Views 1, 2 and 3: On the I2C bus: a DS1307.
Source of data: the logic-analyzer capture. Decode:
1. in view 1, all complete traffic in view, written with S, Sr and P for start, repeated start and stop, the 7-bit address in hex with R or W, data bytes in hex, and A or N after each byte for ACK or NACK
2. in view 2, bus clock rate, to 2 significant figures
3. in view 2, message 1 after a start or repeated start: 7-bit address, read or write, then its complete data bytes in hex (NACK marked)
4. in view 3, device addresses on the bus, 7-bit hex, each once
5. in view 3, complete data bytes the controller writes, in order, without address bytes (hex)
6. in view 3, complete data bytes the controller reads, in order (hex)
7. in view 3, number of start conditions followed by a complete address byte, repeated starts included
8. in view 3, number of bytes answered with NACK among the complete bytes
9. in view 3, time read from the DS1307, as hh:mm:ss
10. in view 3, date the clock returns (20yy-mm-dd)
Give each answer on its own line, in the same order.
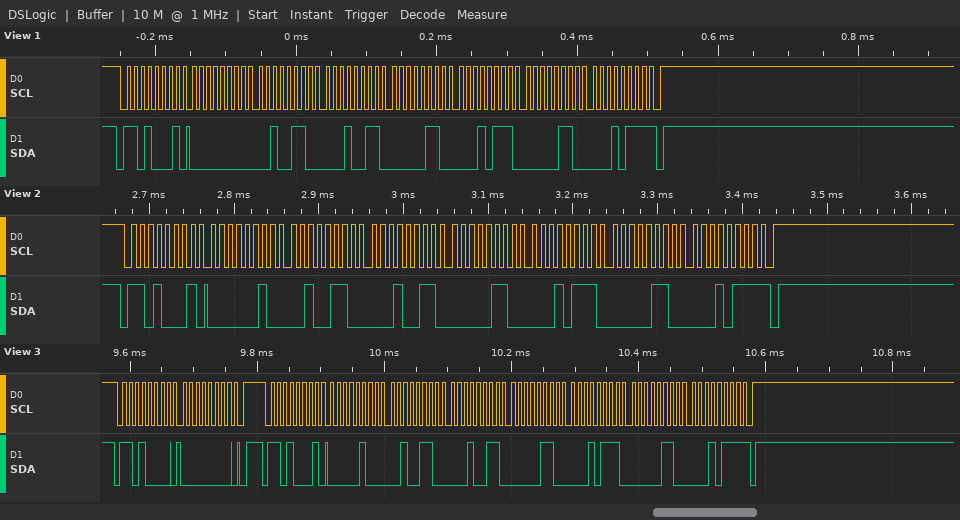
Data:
S 68R A 00 A 26 A 13 A 06 A 17 A 06 A 17 N P
100 kHz
0x68 read: 02 26 13 06 17 06 17 NACK
0x68
00
04 26 13 06 17 06 17
2
1
13:26:04
2017-06-17
